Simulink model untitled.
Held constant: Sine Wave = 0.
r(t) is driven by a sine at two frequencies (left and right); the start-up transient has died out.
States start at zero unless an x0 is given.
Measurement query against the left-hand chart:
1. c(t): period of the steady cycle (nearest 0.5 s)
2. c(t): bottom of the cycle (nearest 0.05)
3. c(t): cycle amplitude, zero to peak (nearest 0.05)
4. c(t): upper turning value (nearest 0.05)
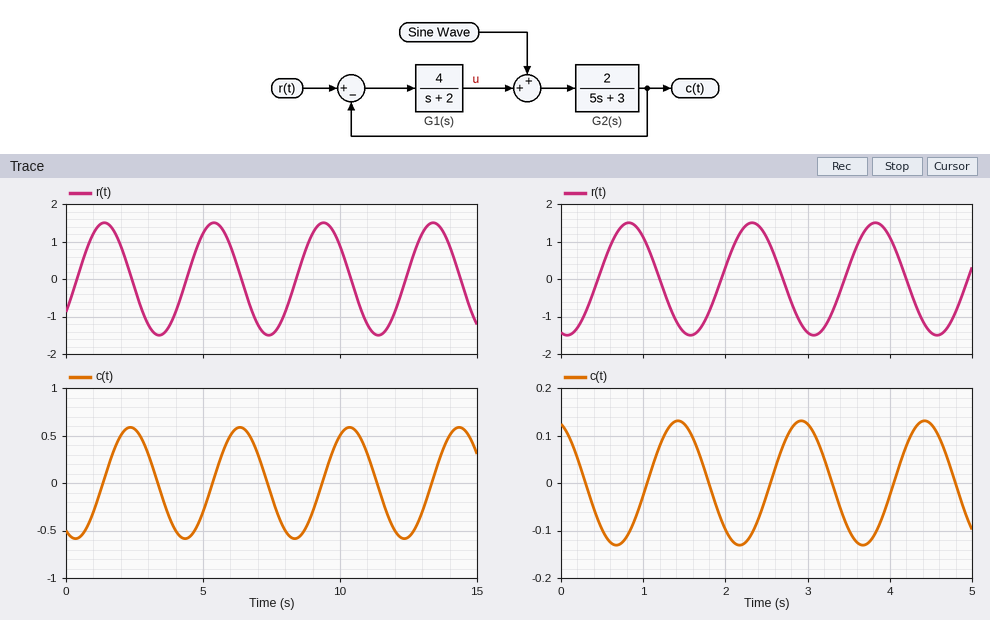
4.0 s
-0.60
0.60
0.60
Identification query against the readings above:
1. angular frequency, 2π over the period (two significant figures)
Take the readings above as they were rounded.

1.6 rad/s
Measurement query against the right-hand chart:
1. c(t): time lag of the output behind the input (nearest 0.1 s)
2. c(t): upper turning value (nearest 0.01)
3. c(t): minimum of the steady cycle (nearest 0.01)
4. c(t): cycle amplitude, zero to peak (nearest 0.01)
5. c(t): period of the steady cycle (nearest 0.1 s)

0.6 s
0.13
-0.13
0.13
1.5 s
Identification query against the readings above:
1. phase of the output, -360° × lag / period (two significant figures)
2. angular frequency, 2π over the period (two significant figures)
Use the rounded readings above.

-140°
4.2 rad/s
